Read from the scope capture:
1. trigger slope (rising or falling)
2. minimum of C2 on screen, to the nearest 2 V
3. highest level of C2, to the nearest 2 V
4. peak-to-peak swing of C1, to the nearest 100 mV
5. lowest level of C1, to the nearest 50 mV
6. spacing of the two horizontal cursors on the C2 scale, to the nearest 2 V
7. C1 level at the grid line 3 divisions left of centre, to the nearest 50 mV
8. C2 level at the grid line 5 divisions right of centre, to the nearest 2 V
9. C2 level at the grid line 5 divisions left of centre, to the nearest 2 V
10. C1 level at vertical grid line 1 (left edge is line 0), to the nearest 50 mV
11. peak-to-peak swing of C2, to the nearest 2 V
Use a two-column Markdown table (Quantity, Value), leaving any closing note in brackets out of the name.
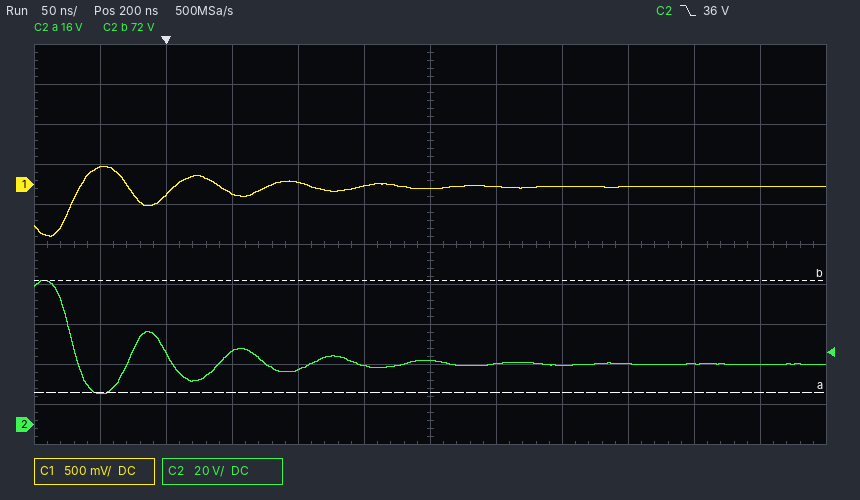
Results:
| Quantity | Value |
|---|---|
| trigger slope | falling |
| minimum of C2 on screen, to the nearest 2 V | 16 V |
| highest level of C2, to the nearest 2 V | 72 V |
| peak-to-peak swing of C1, to the nearest 100 mV | 900 mV |
| lowest level of C1, to the nearest 50 mV | -650 mV |
| spacing of the two horizontal cursors on the C2 scale, to the nearest 2 V | 56 V |
| C1 level at the grid line 3 divisions left of centre, to the nearest 50 mV | -100 mV |
| C2 level at the grid line 5 divisions right of centre, to the nearest 2 V | 30 V |
| C2 level at the grid line 5 divisions left of centre, to the nearest 2 V | 16 V |
| C1 level at vertical grid line 1 (left edge is line 0), to the nearest 50 mV | 200 mV |
| peak-to-peak swing of C2, to the nearest 2 V | 56 V |
